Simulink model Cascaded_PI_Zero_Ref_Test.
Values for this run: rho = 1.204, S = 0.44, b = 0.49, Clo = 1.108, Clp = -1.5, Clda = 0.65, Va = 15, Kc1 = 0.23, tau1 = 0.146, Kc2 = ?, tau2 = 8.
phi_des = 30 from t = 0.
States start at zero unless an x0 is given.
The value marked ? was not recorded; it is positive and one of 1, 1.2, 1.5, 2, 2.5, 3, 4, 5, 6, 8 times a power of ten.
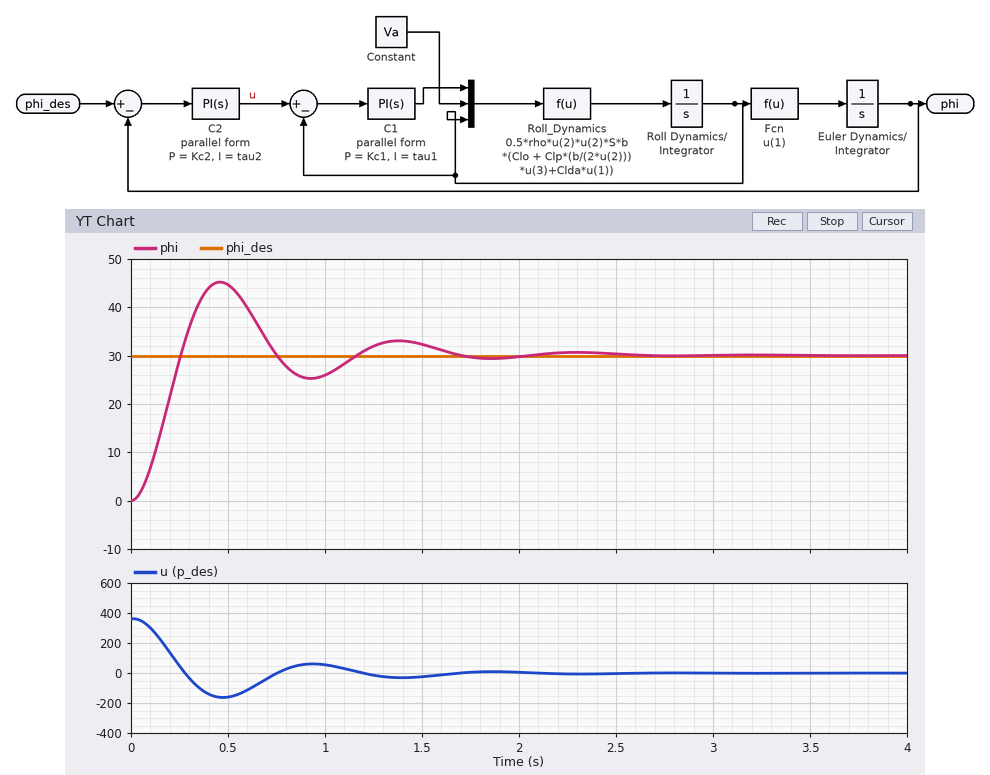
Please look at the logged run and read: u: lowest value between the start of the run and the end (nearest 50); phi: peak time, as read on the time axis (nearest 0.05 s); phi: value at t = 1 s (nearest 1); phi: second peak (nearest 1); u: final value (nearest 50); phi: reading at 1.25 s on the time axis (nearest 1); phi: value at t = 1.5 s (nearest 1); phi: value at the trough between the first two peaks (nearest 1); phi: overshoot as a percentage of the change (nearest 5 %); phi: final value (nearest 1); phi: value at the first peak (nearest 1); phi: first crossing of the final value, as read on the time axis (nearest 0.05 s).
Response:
-150
0.45 s
26
33
0
32
32
25
50 %
30
45
0.25 s
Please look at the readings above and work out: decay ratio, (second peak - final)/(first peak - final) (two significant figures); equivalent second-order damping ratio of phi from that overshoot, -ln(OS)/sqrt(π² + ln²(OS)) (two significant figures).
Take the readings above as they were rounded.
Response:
0.20
0.22
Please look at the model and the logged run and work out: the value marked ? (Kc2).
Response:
12
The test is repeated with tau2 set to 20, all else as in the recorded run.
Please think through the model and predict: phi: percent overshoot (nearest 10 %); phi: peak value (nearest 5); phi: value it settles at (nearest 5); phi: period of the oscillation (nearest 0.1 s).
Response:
70 %
50
30
0.9 s
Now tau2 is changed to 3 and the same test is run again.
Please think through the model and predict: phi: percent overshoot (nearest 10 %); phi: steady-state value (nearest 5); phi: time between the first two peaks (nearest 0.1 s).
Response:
40 %
30
0.9 s
